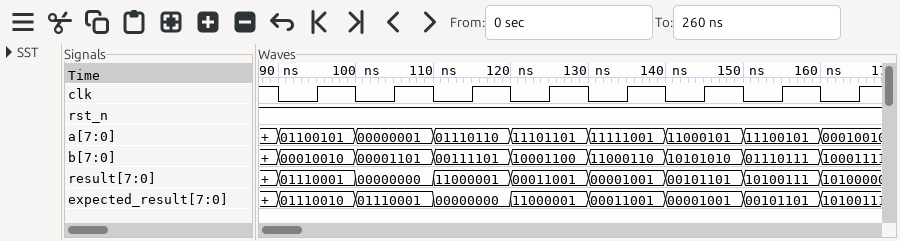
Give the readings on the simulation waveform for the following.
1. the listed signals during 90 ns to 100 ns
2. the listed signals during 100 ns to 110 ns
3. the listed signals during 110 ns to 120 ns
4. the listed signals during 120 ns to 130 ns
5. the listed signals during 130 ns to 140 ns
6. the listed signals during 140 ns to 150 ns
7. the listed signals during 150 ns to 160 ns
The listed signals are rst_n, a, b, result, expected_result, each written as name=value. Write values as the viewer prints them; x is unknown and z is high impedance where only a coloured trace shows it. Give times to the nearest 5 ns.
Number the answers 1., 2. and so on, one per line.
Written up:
1. rst_n=1, a=01100101, b=00010010, result=01110001, expected_result=01110010
2. rst_n=1, a=00000001, b=00001101, result=00000000, expected_result=01110001
3. rst_n=1, a=01110110, b=00111101, result=11000001, expected_result=00000000
4. rst_n=1, a=11101101, b=10001100, result=00011001, expected_result=11000001
5. rst_n=1, a=11111001, b=11000110, result=00001001, expected_result=00011001
6. rst_n=1, a=11000101, b=10101010, result=00101101, expected_result=00001001
7. rst_n=1, a=11100101, b=01110111, result=10100111, expected_result=00101101
